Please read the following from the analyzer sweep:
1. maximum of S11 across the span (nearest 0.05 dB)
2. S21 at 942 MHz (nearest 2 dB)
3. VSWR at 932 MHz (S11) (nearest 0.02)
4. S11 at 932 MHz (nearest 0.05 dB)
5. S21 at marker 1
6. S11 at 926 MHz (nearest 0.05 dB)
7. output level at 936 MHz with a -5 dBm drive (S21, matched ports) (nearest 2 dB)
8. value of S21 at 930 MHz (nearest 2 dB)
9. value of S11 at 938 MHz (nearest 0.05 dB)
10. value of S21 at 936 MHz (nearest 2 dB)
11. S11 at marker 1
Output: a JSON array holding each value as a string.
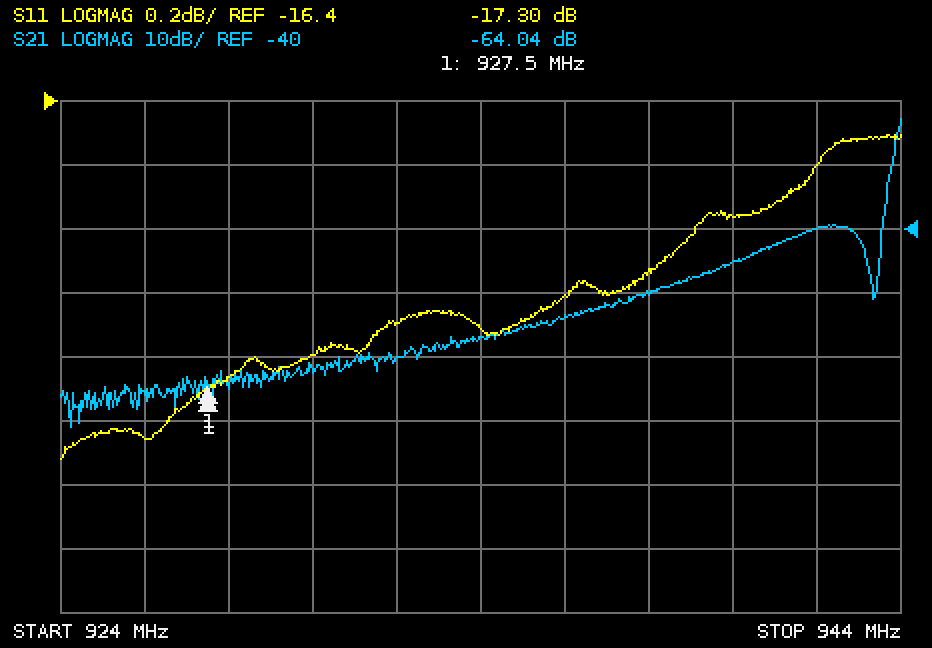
["-16.50 dB", "-40 dB", "1.32", "-17.10 dB", "-64.04 dB", "-17.45 dB", "-58 dBm", "-62 dB", "-16.95 dB", "-54 dB", "-17.30 dB"]
